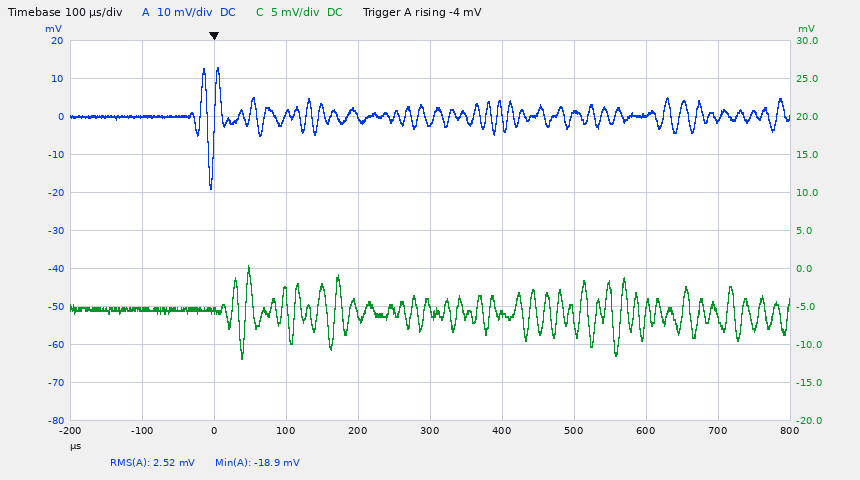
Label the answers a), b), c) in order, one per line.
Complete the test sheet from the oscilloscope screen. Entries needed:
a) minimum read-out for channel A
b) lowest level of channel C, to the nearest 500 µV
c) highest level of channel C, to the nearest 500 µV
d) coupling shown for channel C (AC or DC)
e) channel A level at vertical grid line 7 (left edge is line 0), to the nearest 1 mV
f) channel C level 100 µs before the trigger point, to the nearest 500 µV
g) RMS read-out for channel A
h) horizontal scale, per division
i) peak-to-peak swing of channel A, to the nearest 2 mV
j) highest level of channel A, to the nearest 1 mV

a) -18.9 mV
b) -12.0 mV
c) 500 µV
d) DC
e) 1 mV
f) -5.5 mV
g) 2.52 mV
h) 100 µs
i) 32 mV
j) 13 mV
